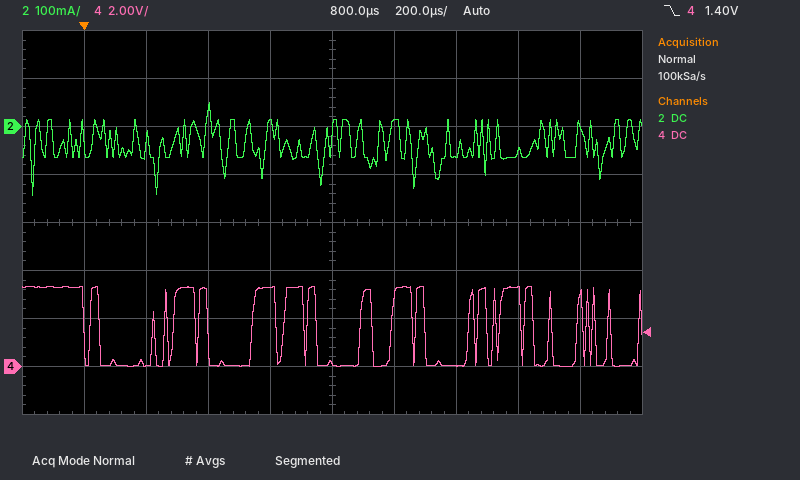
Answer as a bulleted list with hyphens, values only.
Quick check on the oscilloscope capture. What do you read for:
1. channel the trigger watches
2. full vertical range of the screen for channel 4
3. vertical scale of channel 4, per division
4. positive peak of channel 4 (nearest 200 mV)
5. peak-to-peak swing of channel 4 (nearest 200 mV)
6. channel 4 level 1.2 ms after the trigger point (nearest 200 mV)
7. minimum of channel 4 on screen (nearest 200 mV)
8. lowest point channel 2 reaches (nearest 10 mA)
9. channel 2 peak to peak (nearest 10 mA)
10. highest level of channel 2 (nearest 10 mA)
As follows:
- channel 4
- 16 V
- 2 V
- 3.4 V
- 3.4 V
- 0.0 V
- 0.0 V
- -140 mA
- 190 mA
- 50 mA
